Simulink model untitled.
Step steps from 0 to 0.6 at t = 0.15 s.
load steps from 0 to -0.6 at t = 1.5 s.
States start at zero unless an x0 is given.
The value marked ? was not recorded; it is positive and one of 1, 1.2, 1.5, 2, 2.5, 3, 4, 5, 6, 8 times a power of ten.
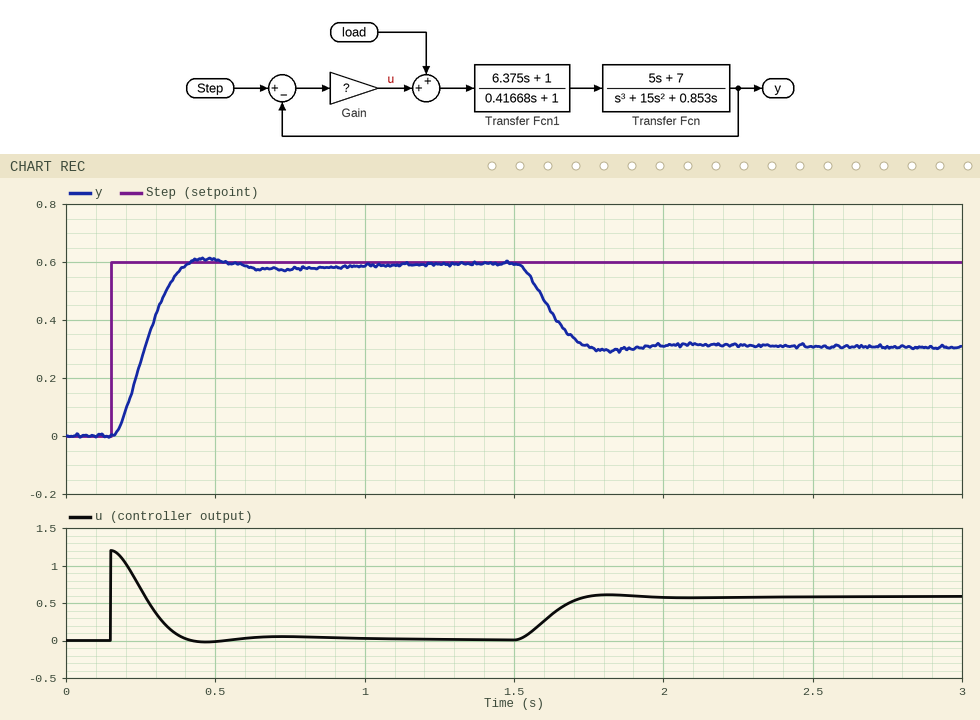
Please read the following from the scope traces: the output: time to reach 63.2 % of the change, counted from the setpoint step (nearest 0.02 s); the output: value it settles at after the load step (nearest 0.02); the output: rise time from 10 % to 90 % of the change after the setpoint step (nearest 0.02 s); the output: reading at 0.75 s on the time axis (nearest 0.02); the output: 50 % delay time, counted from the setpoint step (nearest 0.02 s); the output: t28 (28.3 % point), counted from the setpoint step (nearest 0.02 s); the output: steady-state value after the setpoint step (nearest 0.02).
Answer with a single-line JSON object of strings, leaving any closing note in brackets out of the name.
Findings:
{"the output: time to reach 63.2 % of the change, counted from the setpoint step": "0.14 s", "the output: value it settles at after the load step": "0.30", "the output: rise time from 10 % to 90 % of the change after the setpoint step": "0.16 s", "the output: reading at 0.75 s on the time axis": "0.58", "the output: 50 % delay time, counted from the setpoint step": "0.12 s", "the output: t28 (28.3 % point), counted from the setpoint step": "0.08 s", "the output: steady-state value after the setpoint step": "0.60"}
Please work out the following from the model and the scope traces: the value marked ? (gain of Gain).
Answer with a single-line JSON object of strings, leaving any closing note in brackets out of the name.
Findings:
{"the value marked ?": "2"}
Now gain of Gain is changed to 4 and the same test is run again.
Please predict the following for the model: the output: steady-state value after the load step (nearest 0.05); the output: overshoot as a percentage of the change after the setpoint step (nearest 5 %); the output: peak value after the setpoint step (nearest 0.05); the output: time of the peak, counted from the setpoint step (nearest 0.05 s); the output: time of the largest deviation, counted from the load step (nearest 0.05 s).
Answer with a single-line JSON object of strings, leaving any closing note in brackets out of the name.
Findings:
{"the output: steady-state value after the load step": "0.45", "the output: overshoot as a percentage of the change after the setpoint step": "15 %", "the output: peak value after the setpoint step": "0.70", "the output: time of the peak, counted from the setpoint step": "0.20 s", "the output: time of the largest deviation, counted from the load step": "0.20 s"}
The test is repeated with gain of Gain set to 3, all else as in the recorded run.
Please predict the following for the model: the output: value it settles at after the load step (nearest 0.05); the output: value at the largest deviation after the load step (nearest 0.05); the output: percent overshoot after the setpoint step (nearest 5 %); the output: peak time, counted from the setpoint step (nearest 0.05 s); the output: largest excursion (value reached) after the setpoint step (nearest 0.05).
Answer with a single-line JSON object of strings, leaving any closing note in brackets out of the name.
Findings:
{"the output: value it settles at after the load step": "0.40", "the output: value at the largest deviation after the load step": "0.40", "the output: percent overshoot after the setpoint step": "10 %", "the output: peak time, counted from the setpoint step": "0.25 s", "the output: largest excursion (value reached) after the setpoint step": "0.65"}
